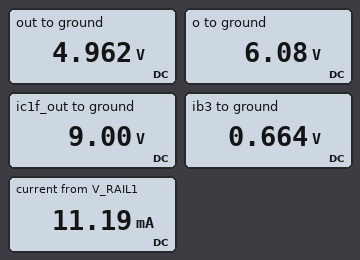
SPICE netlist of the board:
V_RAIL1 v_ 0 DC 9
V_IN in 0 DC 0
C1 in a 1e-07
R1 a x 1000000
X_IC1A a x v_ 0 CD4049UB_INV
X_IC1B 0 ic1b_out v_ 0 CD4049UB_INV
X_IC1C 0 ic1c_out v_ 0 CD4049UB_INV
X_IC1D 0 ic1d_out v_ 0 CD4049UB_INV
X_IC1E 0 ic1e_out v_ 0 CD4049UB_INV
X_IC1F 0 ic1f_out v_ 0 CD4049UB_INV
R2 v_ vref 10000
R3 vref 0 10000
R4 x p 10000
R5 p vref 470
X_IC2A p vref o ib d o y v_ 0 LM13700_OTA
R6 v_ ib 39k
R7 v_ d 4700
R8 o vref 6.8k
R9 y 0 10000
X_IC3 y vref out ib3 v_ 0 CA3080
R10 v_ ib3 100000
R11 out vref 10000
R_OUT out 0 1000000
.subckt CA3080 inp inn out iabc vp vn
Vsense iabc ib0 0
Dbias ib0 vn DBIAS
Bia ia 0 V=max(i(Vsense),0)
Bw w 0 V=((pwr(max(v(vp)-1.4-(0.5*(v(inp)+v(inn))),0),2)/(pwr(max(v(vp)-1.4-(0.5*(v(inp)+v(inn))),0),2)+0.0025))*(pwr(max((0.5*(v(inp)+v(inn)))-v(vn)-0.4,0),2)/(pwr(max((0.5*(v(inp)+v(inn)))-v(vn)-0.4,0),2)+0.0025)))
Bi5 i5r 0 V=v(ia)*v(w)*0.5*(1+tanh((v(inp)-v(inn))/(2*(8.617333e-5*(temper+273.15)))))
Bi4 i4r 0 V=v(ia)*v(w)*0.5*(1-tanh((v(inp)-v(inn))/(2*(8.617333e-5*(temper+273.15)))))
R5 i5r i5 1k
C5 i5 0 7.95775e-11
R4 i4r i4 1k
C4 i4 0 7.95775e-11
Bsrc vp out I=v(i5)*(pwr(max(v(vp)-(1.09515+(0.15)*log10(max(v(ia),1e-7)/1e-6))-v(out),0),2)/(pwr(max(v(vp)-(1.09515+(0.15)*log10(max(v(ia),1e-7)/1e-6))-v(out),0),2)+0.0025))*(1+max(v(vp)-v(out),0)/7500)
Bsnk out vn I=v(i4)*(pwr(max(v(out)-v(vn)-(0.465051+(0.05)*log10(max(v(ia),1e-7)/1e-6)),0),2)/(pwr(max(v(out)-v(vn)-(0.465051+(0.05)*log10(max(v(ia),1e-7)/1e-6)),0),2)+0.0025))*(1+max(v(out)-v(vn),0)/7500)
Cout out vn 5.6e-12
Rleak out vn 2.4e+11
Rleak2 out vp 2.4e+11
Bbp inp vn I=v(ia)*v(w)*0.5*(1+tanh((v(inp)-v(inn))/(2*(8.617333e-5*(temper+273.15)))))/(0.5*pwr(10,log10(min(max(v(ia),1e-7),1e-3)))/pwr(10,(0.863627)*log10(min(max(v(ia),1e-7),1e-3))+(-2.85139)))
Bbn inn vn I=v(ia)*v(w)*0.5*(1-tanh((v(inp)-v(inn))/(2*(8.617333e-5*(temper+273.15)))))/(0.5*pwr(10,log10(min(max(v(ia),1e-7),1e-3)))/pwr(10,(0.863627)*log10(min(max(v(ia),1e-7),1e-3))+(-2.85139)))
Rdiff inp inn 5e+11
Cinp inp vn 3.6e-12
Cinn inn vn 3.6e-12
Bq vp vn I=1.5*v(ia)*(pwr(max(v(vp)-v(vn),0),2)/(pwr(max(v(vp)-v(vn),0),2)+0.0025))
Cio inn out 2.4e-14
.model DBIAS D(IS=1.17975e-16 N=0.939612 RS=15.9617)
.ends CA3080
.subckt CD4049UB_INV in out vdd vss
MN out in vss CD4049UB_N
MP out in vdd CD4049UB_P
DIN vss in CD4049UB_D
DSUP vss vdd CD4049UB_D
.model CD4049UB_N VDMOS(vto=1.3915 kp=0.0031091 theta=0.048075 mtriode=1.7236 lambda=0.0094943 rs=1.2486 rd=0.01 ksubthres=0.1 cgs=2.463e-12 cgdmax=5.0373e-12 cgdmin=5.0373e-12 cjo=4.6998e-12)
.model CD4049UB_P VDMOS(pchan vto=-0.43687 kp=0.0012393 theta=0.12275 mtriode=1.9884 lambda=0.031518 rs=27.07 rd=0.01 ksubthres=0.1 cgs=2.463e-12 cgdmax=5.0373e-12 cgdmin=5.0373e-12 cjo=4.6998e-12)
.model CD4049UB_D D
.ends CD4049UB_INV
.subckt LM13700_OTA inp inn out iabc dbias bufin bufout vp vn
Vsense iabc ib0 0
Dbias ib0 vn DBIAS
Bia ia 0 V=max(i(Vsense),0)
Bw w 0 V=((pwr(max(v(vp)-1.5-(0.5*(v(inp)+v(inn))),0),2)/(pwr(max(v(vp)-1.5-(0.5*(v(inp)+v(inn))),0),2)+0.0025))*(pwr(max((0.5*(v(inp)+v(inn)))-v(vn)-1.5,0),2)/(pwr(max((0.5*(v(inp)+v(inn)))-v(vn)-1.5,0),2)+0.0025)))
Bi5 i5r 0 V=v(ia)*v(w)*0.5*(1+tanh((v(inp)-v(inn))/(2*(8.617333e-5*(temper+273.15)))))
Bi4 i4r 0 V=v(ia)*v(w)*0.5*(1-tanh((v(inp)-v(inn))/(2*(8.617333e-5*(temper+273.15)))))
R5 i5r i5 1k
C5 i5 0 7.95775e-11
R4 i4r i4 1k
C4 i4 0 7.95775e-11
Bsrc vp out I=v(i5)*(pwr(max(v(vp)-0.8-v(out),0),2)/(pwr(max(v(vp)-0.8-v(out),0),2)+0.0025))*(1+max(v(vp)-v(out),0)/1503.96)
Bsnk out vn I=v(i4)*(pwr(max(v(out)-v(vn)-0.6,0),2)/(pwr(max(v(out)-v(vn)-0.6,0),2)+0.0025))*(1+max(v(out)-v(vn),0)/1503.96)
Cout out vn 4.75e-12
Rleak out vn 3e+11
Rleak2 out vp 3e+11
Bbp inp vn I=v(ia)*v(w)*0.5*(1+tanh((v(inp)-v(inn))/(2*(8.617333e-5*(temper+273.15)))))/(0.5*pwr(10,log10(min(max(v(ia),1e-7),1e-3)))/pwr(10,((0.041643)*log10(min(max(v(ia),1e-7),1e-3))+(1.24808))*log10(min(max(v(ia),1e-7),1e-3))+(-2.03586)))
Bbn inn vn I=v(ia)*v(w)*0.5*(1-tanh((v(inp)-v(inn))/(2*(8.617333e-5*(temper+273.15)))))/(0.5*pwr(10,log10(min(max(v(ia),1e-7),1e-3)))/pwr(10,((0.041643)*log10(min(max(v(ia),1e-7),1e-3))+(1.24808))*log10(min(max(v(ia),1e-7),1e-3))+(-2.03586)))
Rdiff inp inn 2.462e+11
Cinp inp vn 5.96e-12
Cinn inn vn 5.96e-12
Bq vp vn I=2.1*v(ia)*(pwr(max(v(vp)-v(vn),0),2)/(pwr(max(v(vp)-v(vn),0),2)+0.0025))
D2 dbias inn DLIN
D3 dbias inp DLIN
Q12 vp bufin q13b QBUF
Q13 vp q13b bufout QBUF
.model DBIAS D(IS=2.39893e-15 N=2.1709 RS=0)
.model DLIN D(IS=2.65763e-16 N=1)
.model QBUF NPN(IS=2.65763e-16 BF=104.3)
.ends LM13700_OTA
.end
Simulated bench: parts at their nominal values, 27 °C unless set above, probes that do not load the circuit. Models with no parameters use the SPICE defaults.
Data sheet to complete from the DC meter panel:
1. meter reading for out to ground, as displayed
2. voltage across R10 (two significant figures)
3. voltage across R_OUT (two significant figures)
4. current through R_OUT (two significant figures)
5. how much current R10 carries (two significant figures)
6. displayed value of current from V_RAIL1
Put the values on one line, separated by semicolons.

4.962 V; 8.3 V; 5.0 V; 5.0 µA; 83 µA; 11.19 mA
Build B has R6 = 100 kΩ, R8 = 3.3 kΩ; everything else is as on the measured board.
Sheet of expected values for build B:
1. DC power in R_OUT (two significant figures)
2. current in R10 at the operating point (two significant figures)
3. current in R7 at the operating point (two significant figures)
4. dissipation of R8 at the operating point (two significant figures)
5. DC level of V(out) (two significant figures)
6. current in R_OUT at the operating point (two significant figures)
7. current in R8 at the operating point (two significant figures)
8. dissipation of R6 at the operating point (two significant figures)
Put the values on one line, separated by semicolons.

24 µW; 83 µA; 530 µA; 730 nW; 4.9 V; 4.9 µA; 15 µA; 580 µW
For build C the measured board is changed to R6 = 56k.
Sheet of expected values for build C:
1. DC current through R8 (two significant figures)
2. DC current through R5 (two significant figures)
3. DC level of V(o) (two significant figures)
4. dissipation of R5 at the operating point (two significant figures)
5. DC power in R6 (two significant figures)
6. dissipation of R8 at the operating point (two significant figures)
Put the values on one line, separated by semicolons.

25 µA; 21 µA; 6.0 V; 200 nW; 1.0 mW; 4.3 µW
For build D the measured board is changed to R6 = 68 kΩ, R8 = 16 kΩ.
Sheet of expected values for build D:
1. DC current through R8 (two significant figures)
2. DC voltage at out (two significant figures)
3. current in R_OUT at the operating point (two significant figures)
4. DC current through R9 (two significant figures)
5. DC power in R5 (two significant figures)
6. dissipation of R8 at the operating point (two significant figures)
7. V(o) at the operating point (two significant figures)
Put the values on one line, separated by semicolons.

21 µA; 4.9 V; 4.9 µA; 480 µA; 210 nW; 7.1 µW; 6.2 V
